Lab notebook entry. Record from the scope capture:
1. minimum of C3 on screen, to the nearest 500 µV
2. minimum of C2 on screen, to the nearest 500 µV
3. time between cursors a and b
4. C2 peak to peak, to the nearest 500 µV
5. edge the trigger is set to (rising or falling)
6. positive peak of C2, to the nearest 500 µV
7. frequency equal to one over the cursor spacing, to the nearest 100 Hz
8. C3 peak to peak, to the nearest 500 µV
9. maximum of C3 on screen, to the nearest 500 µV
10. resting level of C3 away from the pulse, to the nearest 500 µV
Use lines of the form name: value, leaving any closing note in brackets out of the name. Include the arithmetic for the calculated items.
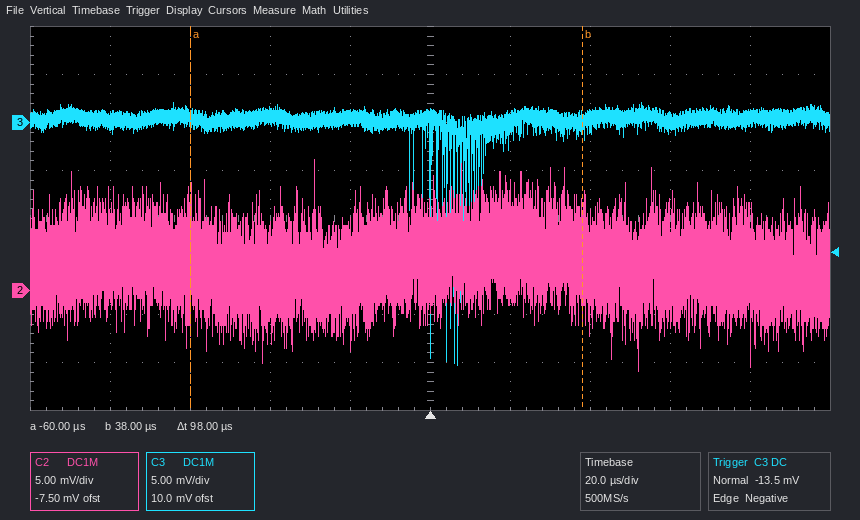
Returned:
minimum of C3 on screen, to the nearest 500 µV: -25.5 mV
minimum of C2 on screen, to the nearest 500 µV: -8.5 mV
time between cursors a and b: 98 µs
C2 peak to peak, to the nearest 500 µV: 13.5 mV − (-8.5 mV) = 22.0 mV
edge the trigger is set to: falling
positive peak of C2, to the nearest 500 µV: 13.5 mV
frequency equal to one over the cursor spacing, to the nearest 100 Hz: 1 / 98 µs ≈ 10.2 kHz
C3 peak to peak, to the nearest 500 µV: 2.0 mV − (-25.5 mV) = 27.5 mV
maximum of C3 on screen, to the nearest 500 µV: 2.0 mV
resting level of C3 away from the pulse, to the nearest 500 µV: 500 µV
